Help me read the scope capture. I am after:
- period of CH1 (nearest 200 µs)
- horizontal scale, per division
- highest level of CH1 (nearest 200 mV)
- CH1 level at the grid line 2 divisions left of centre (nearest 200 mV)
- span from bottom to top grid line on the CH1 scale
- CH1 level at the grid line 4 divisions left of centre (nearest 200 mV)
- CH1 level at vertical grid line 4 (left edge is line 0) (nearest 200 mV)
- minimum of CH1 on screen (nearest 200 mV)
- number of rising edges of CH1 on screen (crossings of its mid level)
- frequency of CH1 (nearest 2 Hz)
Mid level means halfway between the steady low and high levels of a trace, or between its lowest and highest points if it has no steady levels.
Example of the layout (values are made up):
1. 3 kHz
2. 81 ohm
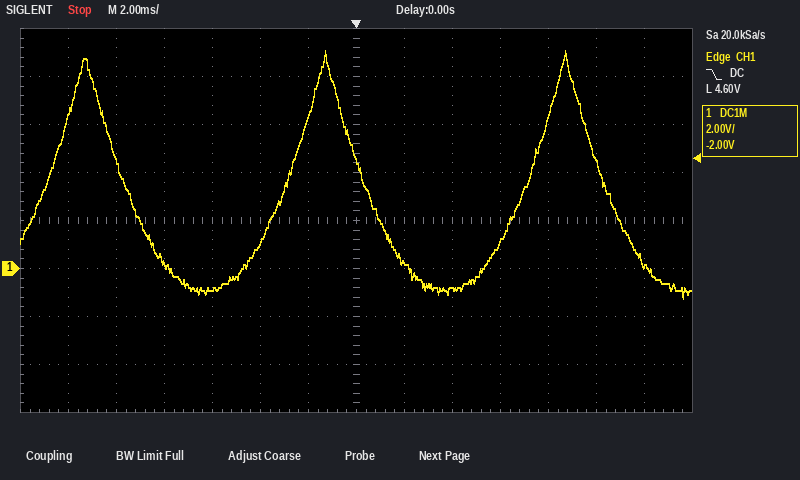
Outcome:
1. 10.0 ms
2. 2 ms
3. 9.0 V
4. 1.0 V
5. 16 V
6. 200 mV
7. -800 mV
8. -1.2 V
9. 3
10. 100 Hz
